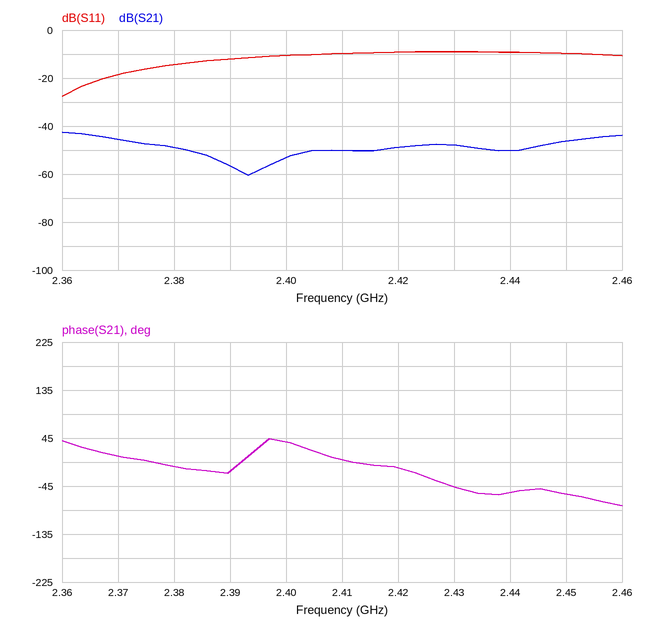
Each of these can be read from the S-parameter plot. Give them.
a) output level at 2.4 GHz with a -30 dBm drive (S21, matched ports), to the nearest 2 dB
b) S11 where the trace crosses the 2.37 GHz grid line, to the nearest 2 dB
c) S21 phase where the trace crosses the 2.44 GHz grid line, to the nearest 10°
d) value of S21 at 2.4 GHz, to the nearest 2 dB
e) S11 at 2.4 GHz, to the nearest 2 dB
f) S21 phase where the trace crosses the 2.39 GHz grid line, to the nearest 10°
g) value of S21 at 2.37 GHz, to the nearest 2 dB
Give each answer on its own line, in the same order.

-84 dBm
-18 dB
-60°
-54 dB
-10 dB
-20°
-46 dB
